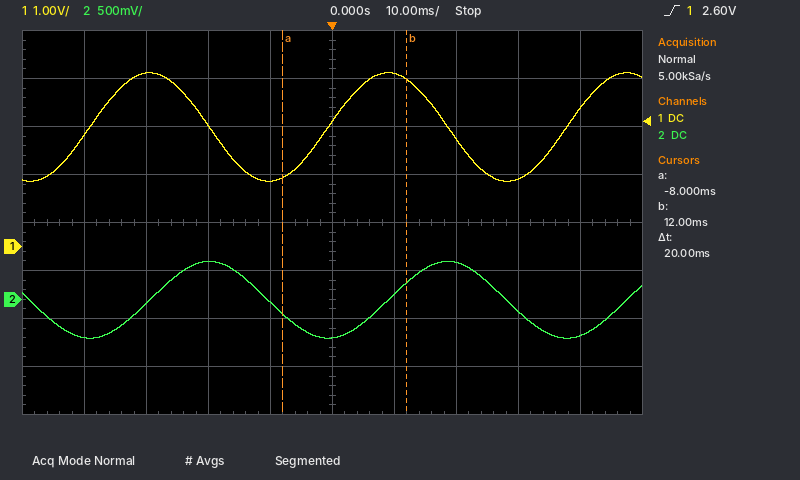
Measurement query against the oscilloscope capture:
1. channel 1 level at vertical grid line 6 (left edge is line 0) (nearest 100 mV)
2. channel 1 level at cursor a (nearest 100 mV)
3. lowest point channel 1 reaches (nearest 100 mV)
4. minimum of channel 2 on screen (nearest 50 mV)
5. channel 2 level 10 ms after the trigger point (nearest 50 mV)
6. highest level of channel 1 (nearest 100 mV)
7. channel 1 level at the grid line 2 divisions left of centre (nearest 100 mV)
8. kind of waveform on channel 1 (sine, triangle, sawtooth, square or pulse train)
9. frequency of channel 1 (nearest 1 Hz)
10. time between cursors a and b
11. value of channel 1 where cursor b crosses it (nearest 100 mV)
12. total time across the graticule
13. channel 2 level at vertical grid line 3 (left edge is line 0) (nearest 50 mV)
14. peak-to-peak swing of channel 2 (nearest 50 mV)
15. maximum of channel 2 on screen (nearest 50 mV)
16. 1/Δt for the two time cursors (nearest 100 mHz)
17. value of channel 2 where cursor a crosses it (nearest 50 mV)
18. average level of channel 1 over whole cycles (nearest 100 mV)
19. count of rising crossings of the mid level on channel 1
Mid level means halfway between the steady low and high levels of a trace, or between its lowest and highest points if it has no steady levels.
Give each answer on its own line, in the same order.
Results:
3.6 V
1.4 V
1.4 V
-400 mV
50 mV
3.6 V
2.5 V
sine
26 Hz
20 ms
3.5 V
100 ms
400 mV
800 mV
400 mV
50.0 Hz
-150 mV
2.5 V
3
